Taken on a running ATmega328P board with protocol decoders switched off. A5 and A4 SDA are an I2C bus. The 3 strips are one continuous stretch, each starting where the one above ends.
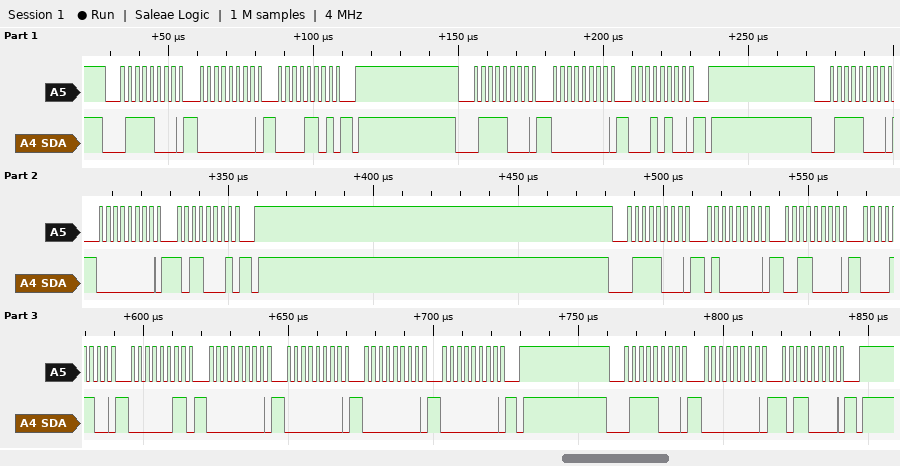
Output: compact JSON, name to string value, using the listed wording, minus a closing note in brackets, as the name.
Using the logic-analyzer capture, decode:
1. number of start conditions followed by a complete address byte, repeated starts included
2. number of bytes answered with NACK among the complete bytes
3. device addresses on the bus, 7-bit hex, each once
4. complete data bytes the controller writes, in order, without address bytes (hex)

{"number of start conditions followed by a complete address byte, repeated starts included": "5", "number of bytes answered with NACK among the complete bytes": "0", "device addresses on the bus, 7-bit hex, each once": "0x3C", "complete data bytes the controller writes, in order, without address bytes": "00 0D 00 14 00 B1 40 30 0C 03 00 00 00 00 00 B0"}
